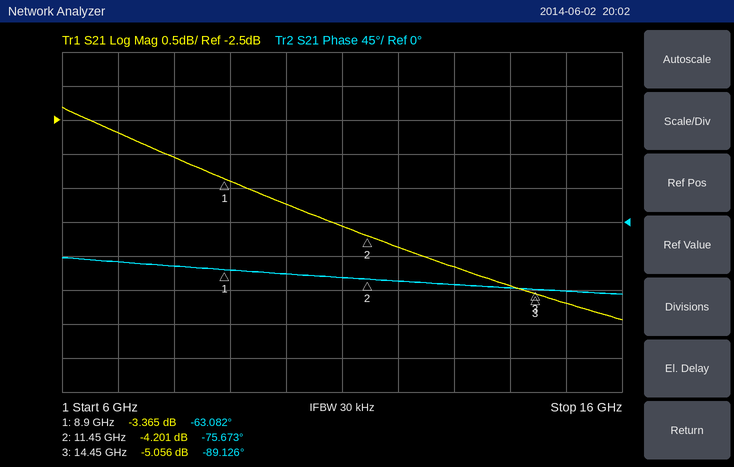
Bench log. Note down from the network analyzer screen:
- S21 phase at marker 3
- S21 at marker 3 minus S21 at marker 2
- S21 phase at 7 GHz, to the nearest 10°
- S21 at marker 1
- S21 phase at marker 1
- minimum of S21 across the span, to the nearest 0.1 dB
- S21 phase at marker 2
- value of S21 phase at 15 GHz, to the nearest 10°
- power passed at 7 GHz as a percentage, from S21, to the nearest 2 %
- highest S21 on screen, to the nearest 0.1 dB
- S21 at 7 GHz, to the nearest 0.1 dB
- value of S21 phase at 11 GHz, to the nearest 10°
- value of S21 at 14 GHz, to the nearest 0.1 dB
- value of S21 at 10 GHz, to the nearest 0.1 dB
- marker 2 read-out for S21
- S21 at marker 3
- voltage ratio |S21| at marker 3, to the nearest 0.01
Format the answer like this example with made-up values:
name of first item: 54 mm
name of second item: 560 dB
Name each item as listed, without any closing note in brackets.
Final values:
S21 phase at marker 3: -89.126°
S21 at marker 3 minus S21 at marker 2: -0.855 dB
S21 phase at 7 GHz, to the nearest 10°: -50°
S21 at marker 1: -3.365 dB
S21 phase at marker 1: -63.082°
minimum of S21 across the span, to the nearest 0.1 dB: -5.4 dB
S21 phase at marker 2: -75.673°
value of S21 phase at 15 GHz, to the nearest 10°: -90°
power passed at 7 GHz as a percentage, from S21, to the nearest 2 %: 54 %
highest S21 on screen, to the nearest 0.1 dB: -2.3 dB
S21 at 7 GHz, to the nearest 0.1 dB: -2.7 dB
value of S21 phase at 11 GHz, to the nearest 10°: -70°
value of S21 at 14 GHz, to the nearest 0.1 dB: -4.9 dB
value of S21 at 10 GHz, to the nearest 0.1 dB: -3.7 dB
marker 2 read-out for S21: -4.201 dB
S21 at marker 3: -5.056 dB
voltage ratio |S21| at marker 3, to the nearest 0.01: 0.56
